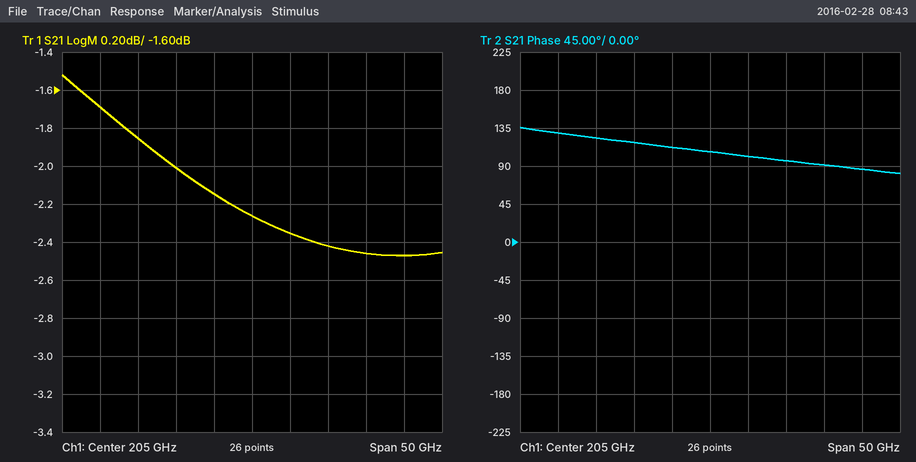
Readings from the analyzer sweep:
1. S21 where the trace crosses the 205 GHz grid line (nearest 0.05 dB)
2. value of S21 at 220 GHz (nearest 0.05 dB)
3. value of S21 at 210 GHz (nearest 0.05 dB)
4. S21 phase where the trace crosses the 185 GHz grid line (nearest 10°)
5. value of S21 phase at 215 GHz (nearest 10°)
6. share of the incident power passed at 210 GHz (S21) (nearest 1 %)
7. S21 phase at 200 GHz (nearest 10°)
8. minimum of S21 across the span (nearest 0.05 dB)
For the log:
-2.25 dB
-2.45 dB
-2.35 dB
130°
100°
58 %
110°
-2.45 dB
